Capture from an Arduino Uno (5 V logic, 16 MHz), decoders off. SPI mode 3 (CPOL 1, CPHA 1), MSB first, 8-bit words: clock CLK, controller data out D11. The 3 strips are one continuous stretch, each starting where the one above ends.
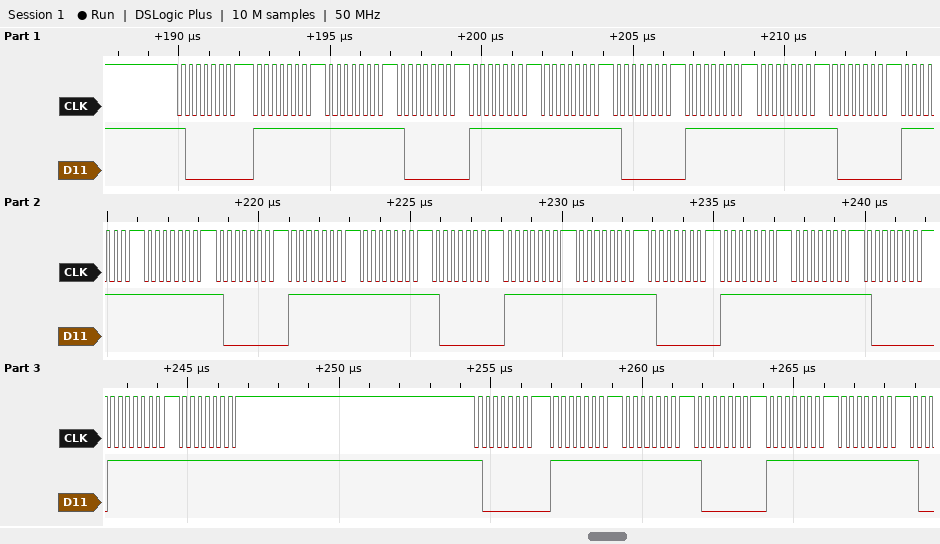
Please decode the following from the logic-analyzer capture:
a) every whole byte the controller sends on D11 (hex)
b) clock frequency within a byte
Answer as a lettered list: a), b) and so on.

a) 80 FF FF 80 FF FF 80 FF FF 80 FF FF 80 FF FF 80 FF FF 80 FF FF 80 FF FF 80 FF FF 80 FF FF
b) 4 MHz
